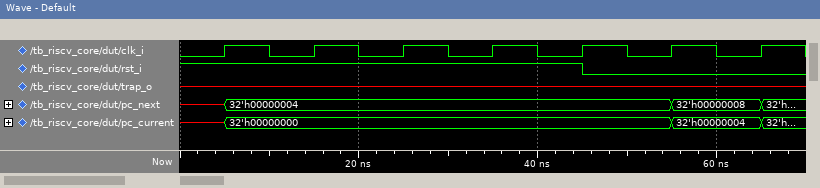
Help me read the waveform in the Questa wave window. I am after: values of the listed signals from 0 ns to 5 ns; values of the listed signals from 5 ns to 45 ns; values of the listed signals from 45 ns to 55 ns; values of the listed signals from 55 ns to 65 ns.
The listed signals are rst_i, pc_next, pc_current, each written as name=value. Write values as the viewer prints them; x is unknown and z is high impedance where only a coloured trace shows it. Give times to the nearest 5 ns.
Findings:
rst_i=1, pc_next=x, pc_current=x
rst_i=1, pc_next=32'h00000004, pc_current=32'h00000000
rst_i=0, pc_next=32'h00000004, pc_current=32'h00000000
rst_i=0, pc_next=32'h00000008, pc_current=32'h00000004
